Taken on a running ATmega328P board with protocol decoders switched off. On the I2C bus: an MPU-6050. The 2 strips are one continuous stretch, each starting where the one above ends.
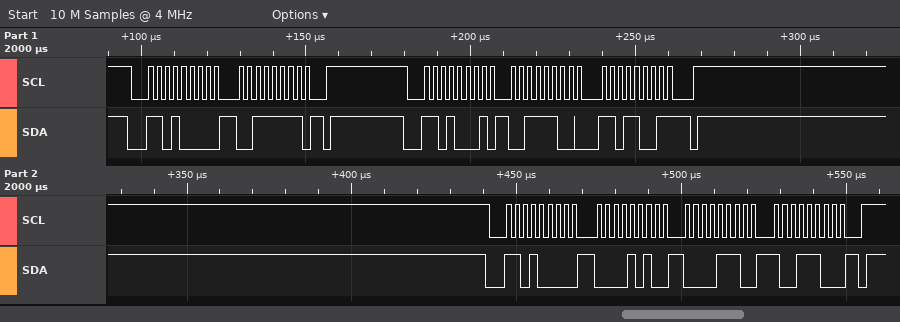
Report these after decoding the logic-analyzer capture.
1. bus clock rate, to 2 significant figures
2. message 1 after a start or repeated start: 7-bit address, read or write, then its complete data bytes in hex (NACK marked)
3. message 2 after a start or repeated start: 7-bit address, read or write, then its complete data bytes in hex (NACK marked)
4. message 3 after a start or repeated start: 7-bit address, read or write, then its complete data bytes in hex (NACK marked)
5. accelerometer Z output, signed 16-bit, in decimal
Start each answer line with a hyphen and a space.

- 400 kHz
- 0x68 write: 3F
- 0x68 read: 3C D9 NACK
- 0x68 write: 0A 0E 9C
- 15577
